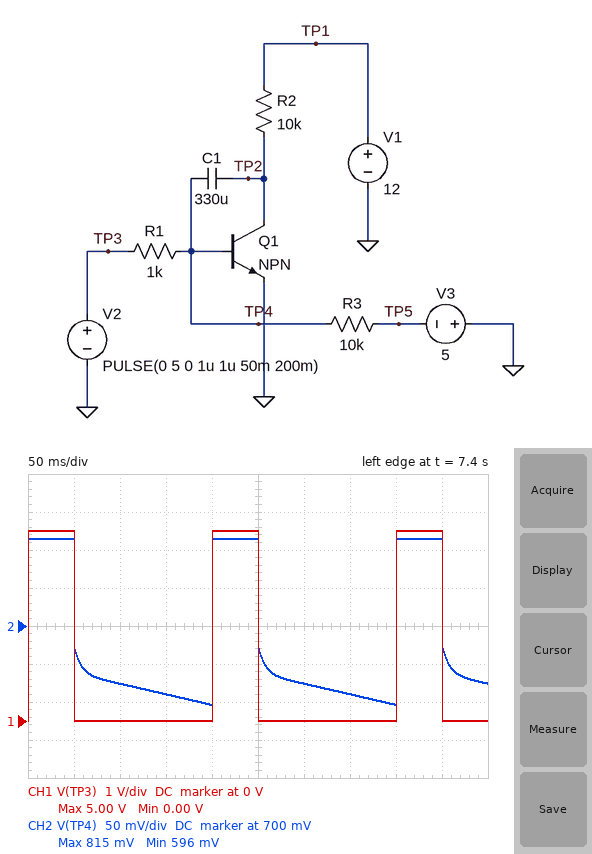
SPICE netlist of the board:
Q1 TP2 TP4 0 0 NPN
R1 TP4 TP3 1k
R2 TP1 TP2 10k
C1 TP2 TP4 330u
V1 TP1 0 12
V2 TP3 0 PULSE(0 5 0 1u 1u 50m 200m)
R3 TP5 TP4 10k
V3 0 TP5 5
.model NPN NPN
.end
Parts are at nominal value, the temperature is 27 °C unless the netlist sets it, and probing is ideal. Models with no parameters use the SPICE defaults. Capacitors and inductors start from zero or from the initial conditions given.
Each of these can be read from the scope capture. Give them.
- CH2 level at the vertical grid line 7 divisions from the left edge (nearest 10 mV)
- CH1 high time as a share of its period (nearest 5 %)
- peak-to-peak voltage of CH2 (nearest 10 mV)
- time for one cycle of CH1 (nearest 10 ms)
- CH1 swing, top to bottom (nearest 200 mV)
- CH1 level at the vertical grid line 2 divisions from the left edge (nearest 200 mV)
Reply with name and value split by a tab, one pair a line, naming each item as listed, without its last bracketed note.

CH2 level at the vertical grid line 7 divisions from the left edge	610 mV
CH1 high time as a share of its period	25 %
peak-to-peak voltage of CH2	220 mV
time for one cycle of CH1	200 ms
CH1 swing, top to bottom	5.0 V
CH1 level at the vertical grid line 2 divisions from the left edge	0 V
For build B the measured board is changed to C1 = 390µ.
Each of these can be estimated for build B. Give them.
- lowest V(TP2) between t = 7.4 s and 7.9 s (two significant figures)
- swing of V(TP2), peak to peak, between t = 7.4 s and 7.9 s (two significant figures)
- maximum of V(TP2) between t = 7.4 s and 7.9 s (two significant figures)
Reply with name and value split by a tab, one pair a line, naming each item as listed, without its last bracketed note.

lowest V(TP2) between t = 7.4 s and 7.9 s	-16 mV
swing of V(TP2), peak to peak, between t = 7.4 s and 7.9 s	630 mV
maximum of V(TP2) between t = 7.4 s and 7.9 s	620 mV
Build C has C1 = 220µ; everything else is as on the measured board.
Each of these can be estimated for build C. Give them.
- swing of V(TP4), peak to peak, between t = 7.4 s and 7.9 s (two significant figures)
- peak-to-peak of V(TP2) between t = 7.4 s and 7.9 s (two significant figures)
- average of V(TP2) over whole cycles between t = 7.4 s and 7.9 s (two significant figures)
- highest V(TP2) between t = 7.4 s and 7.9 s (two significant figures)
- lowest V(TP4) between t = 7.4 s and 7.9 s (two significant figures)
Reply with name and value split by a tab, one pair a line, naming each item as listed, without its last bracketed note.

swing of V(TP4), peak to peak, between t = 7.4 s and 7.9 s	240 mV
peak-to-peak of V(TP2) between t = 7.4 s and 7.9 s	910 mV
average of V(TP2) over whole cycles between t = 7.4 s and 7.9 s	330 mV
highest V(TP2) between t = 7.4 s and 7.9 s	880 mV
lowest V(TP4) between t = 7.4 s and 7.9 s	580 mV
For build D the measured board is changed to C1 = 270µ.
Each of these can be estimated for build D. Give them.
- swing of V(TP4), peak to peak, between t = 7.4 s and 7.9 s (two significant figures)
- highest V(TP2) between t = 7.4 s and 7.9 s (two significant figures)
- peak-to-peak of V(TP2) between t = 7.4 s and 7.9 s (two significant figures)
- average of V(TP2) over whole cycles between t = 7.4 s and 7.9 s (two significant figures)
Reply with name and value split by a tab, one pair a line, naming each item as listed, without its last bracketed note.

swing of V(TP4), peak to peak, between t = 7.4 s and 7.9 s	230 mV
highest V(TP2) between t = 7.4 s and 7.9 s	750 mV
peak-to-peak of V(TP2) between t = 7.4 s and 7.9 s	780 mV
average of V(TP2) over whole cycles between t = 7.4 s and 7.9 s	270 mV
